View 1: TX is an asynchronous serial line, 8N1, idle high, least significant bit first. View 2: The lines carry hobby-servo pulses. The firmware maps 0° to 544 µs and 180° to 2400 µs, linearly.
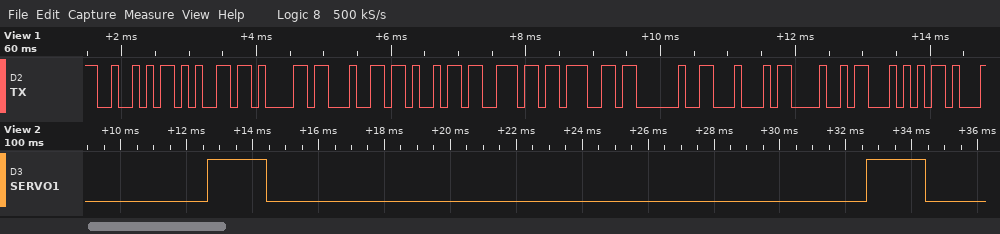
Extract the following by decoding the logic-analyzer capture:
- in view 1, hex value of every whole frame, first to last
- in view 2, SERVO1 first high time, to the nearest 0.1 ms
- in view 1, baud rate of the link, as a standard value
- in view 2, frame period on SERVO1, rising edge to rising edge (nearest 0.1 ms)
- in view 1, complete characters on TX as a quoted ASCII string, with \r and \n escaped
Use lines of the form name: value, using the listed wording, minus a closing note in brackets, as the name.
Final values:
in view 1, hex value of every whole frame, first to last: 0x52 0x65 0x61 0x64 0x69 0x6E 0x67 0x20 0x44 0x48 0x54
in view 2, SERVO1 first high time, to the nearest 0.1 ms: 1.8 ms
in view 1, baud rate of the link, as a standard value: 9600 baud
in view 2, frame period on SERVO1, rising edge to rising edge: 20.0 ms
in view 1, complete characters on TX as a quoted ASCII string, with \r and \n escaped: "Reading DHT"
